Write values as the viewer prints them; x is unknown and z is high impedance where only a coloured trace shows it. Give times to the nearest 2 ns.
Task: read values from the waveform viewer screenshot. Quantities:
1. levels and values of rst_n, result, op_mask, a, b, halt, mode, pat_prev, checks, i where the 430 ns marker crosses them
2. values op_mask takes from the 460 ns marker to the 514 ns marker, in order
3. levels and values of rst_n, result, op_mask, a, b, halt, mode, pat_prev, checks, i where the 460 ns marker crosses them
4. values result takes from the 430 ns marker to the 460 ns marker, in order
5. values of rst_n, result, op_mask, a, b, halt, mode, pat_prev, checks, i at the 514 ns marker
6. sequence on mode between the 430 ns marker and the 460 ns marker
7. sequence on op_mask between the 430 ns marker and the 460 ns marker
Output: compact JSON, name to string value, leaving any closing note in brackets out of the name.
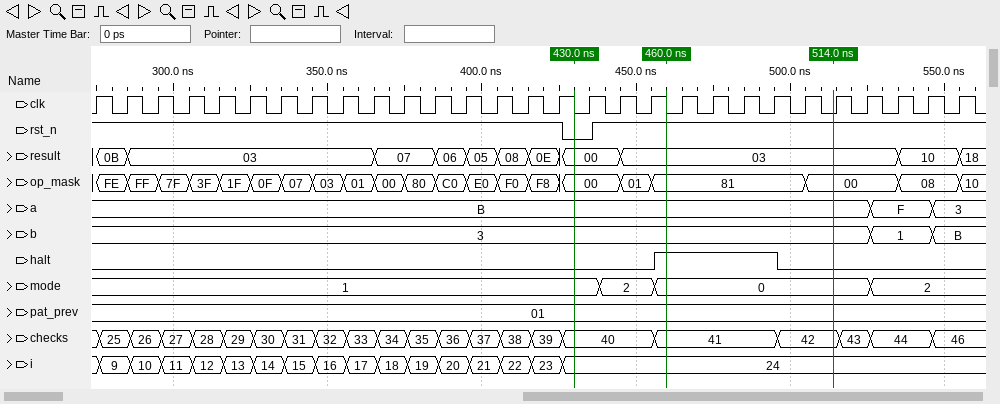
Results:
{"levels and values of rst_n, result, op_mask, a, b, halt, mode, pat_prev, checks, i where the 430 ns marker crosses them": "rst_n=0, result=00, op_mask=00, a=B, b=3, halt=0, mode=1, pat_prev=01, checks=40, i=24", "values op_mask takes from the 460 ns marker to the 514 ns marker, in order": "81, 00", "levels and values of rst_n, result, op_mask, a, b, halt, mode, pat_prev, checks, i where the 460 ns marker crosses them": "rst_n=1, result=03, op_mask=81, a=B, b=3, halt=1, mode=0, pat_prev=01, checks=41, i=24", "values result takes from the 430 ns marker to the 460 ns marker, in order": "00, 03", "values of rst_n, result, op_mask, a, b, halt, mode, pat_prev, checks, i at the 514 ns marker": "rst_n=1, result=03, op_mask=00, a=B, b=3, halt=0, mode=0, pat_prev=01, checks=42, i=24", "sequence on mode between the 430 ns marker and the 460 ns marker": "1, 2, 0", "sequence on op_mask between the 430 ns marker and the 460 ns marker": "00, 01, 81"}
